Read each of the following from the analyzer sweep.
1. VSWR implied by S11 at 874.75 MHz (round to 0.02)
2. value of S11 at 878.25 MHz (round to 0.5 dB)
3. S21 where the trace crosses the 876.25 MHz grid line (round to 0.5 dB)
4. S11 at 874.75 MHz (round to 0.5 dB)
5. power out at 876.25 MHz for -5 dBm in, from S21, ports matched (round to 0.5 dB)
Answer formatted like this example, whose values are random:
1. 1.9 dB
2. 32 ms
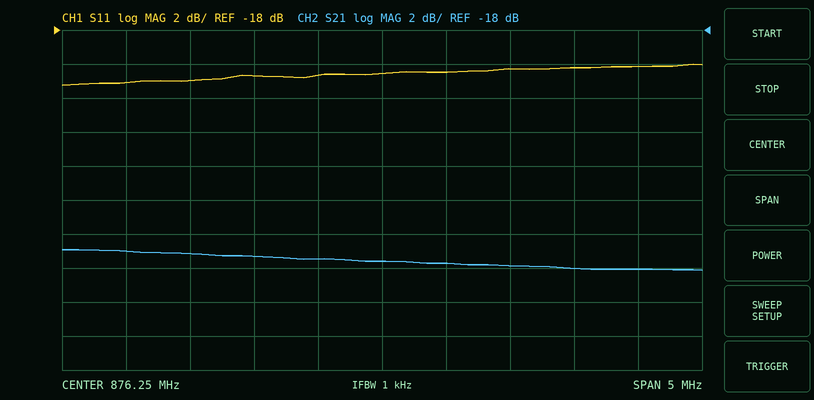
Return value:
1. 1.20
2. -20.0 dB
3. -31.5 dB
4. -21.0 dB
5. -36.5 dBm
